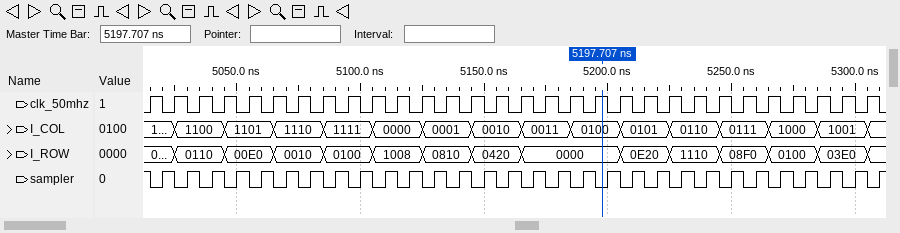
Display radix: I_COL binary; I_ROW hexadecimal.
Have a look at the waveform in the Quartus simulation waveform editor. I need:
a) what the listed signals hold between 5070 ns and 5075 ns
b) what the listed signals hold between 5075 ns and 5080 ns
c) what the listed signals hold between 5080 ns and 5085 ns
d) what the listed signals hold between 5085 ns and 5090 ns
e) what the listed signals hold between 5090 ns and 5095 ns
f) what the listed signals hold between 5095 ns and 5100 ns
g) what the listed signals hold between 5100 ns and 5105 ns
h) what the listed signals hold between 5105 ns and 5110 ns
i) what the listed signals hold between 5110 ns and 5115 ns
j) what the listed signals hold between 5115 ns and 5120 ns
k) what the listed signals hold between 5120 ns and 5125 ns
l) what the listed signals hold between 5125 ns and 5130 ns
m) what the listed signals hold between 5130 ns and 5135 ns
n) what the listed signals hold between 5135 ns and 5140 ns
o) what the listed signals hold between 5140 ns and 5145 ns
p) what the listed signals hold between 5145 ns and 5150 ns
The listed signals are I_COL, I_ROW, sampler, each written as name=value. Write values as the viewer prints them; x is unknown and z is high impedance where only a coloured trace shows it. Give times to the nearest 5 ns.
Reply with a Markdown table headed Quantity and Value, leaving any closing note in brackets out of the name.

| Quantity | Value |
|---|---|
| what the listed signals hold between 5070 ns and 5075 ns | I_COL=1110, I_ROW=0010, sampler=1 |
| what the listed signals hold between 5075 ns and 5080 ns | I_COL=1110, I_ROW=0010, sampler=0 |
| what the listed signals hold between 5080 ns and 5085 ns | I_COL=1110, I_ROW=0010, sampler=1 |
| what the listed signals hold between 5085 ns and 5090 ns | I_COL=1111, I_ROW=0100, sampler=0 |
| what the listed signals hold between 5090 ns and 5095 ns | I_COL=1111, I_ROW=0100, sampler=1 |
| what the listed signals hold between 5095 ns and 5100 ns | I_COL=1111, I_ROW=0100, sampler=0 |
| what the listed signals hold between 5100 ns and 5105 ns | I_COL=1111, I_ROW=0100, sampler=1 |
| what the listed signals hold between 5105 ns and 5110 ns | I_COL=0000, I_ROW=1008, sampler=0 |
| what the listed signals hold between 5110 ns and 5115 ns | I_COL=0000, I_ROW=1008, sampler=1 |
| what the listed signals hold between 5115 ns and 5120 ns | I_COL=0000, I_ROW=1008, sampler=0 |
| what the listed signals hold between 5120 ns and 5125 ns | I_COL=0000, I_ROW=1008, sampler=1 |
| what the listed signals hold between 5125 ns and 5130 ns | I_COL=0001, I_ROW=0810, sampler=0 |
| what the listed signals hold between 5130 ns and 5135 ns | I_COL=0001, I_ROW=0810, sampler=1 |
| what the listed signals hold between 5135 ns and 5140 ns | I_COL=0001, I_ROW=0810, sampler=0 |
| what the listed signals hold between 5140 ns and 5145 ns | I_COL=0001, I_ROW=0810, sampler=1 |
| what the listed signals hold between 5145 ns and 5150 ns | I_COL=0010, I_ROW=0420, sampler=0 |
